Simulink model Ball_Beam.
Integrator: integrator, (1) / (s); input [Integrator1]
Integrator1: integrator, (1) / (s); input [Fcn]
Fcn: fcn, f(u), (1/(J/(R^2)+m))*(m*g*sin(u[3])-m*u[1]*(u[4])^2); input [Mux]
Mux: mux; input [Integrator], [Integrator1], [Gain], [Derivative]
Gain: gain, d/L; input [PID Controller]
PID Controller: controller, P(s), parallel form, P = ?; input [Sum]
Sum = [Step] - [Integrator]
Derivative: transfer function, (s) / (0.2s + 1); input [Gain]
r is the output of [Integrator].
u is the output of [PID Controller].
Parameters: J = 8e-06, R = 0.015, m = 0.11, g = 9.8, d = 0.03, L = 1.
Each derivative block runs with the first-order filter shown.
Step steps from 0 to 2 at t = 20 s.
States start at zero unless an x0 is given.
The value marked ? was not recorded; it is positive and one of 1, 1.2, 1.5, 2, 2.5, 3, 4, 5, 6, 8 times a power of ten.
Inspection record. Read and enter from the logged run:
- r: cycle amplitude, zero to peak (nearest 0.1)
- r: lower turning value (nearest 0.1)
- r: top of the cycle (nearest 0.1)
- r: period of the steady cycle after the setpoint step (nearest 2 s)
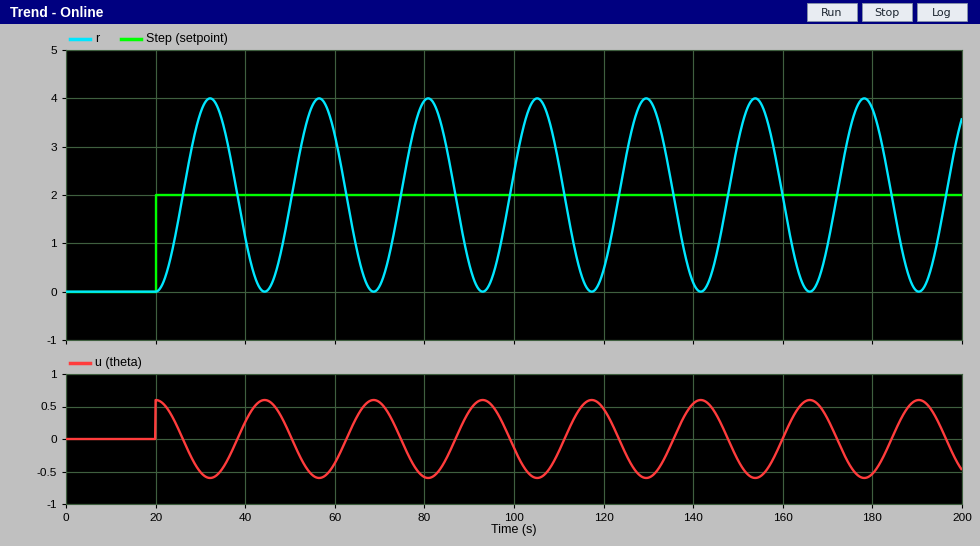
2.0
0.0
4.0
24 s
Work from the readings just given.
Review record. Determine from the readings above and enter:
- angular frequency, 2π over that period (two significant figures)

0.26 rad/s
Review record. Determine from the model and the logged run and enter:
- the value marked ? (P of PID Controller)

0.3
